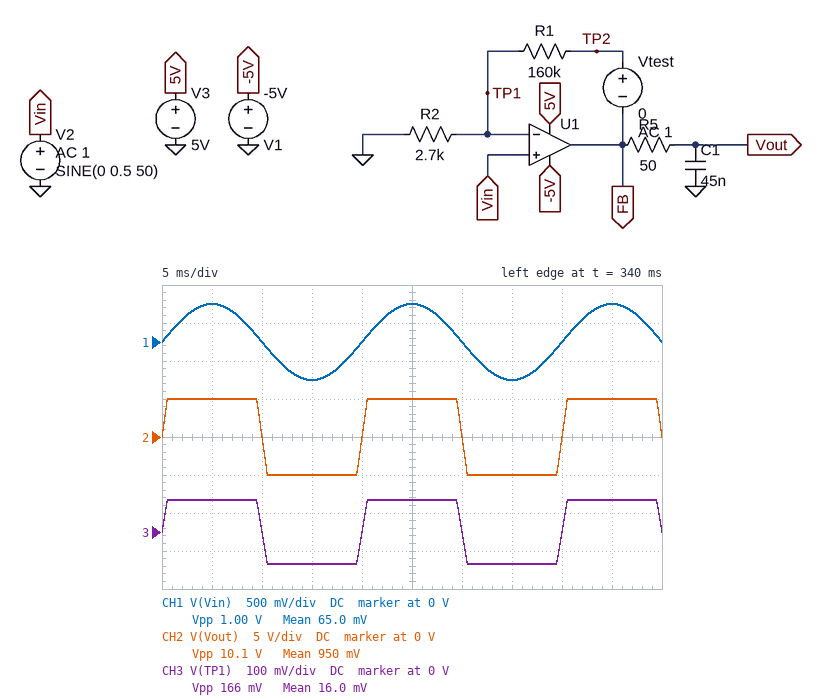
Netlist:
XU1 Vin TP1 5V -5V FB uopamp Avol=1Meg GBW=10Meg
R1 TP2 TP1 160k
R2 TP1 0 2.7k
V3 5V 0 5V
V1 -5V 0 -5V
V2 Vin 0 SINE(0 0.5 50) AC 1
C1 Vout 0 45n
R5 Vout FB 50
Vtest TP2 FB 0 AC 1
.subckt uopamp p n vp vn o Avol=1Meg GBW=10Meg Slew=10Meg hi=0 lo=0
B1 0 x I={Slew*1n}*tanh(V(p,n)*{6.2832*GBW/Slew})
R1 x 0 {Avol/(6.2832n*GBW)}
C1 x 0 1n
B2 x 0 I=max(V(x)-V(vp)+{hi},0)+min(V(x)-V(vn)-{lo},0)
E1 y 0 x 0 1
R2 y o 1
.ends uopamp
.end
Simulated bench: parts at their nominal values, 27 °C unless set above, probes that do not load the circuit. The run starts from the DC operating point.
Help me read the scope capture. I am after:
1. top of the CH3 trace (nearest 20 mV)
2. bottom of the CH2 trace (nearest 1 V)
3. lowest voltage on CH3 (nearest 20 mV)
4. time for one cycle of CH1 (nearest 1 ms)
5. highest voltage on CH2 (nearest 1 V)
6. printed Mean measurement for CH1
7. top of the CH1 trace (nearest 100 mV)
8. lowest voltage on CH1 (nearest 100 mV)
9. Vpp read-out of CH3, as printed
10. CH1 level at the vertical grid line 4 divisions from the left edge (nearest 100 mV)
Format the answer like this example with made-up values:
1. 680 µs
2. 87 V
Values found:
1. 80 mV
2. -5 V
3. -80 mV
4. 20 ms
5. 5 V
6. 65.0 mV
7. 500 mV
8. -500 mV
9. 166 mV
10. 0 V
